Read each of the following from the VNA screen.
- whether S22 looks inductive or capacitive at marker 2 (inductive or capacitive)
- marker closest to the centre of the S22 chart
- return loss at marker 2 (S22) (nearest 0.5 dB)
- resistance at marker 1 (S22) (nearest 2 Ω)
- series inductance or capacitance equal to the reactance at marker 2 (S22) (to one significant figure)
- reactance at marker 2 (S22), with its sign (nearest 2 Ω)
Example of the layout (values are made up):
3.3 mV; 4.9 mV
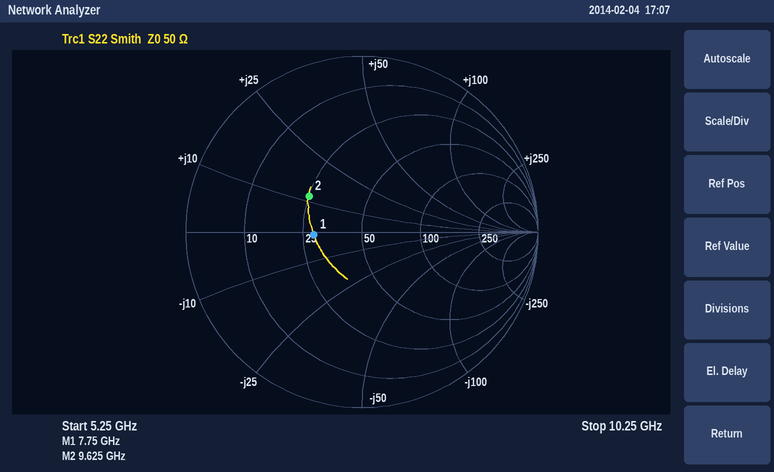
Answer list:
inductive; marker 1; 9.0 dB; 28 Ω; 200 pH; +12 Ω
